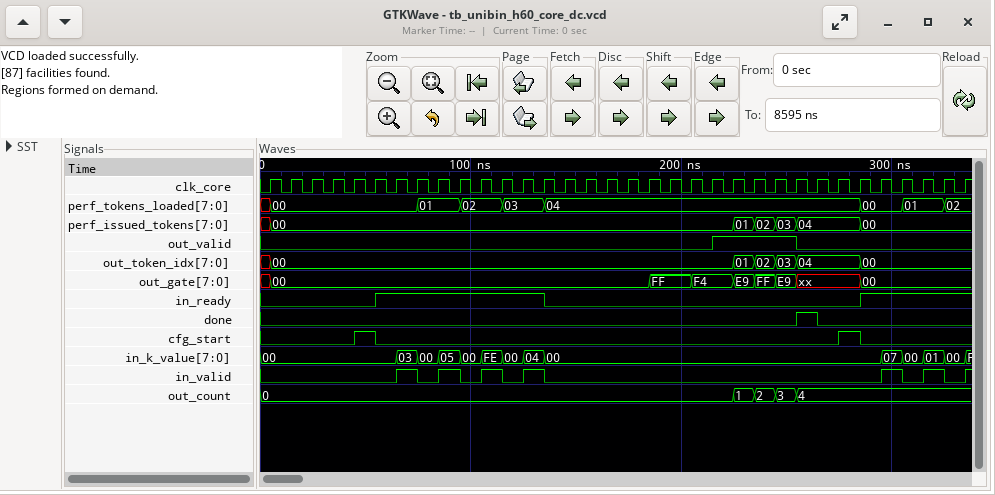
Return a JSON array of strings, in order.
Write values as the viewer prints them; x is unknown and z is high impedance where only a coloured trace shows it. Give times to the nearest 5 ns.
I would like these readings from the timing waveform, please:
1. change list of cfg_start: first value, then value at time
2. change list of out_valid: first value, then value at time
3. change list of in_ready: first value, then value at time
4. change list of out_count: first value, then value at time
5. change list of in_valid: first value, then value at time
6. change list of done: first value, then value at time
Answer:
["0, 1 at 45 ns, 0 at 55 ns, 1 at 275 ns, 0 at 285 ns", "0, 1 at 215 ns, 0 at 255 ns", "0, 1 at 55 ns, 0 at 135 ns, 1 at 285 ns", "0, 1 at 225 ns, 2 at 235 ns, 3 at 245 ns, 4 at 255 ns", "0, 1 at 65 ns, 0 at 75 ns, 1 at 85 ns, 0 at 95 ns, 1 at 105 ns, 0 at 115 ns, 1 at 125 ns, 0 at 135 ns, 1 at 295 ns, 0 at 305 ns, 1 at 315 ns, 0 at 325 ns, 1 at 335 ns", "0, 1 at 255 ns, 0 at 265 ns"]
